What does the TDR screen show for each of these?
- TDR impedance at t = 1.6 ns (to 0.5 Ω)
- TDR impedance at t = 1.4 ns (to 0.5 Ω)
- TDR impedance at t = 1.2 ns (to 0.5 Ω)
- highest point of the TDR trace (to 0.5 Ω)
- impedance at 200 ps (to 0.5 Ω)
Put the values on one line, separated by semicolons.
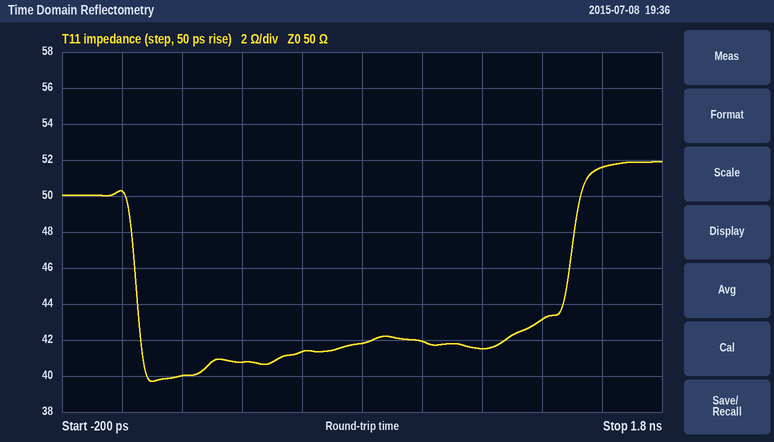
51.5 Ω; 43.0 Ω; 41.5 Ω; 52.0 Ω; 40.0 Ω
